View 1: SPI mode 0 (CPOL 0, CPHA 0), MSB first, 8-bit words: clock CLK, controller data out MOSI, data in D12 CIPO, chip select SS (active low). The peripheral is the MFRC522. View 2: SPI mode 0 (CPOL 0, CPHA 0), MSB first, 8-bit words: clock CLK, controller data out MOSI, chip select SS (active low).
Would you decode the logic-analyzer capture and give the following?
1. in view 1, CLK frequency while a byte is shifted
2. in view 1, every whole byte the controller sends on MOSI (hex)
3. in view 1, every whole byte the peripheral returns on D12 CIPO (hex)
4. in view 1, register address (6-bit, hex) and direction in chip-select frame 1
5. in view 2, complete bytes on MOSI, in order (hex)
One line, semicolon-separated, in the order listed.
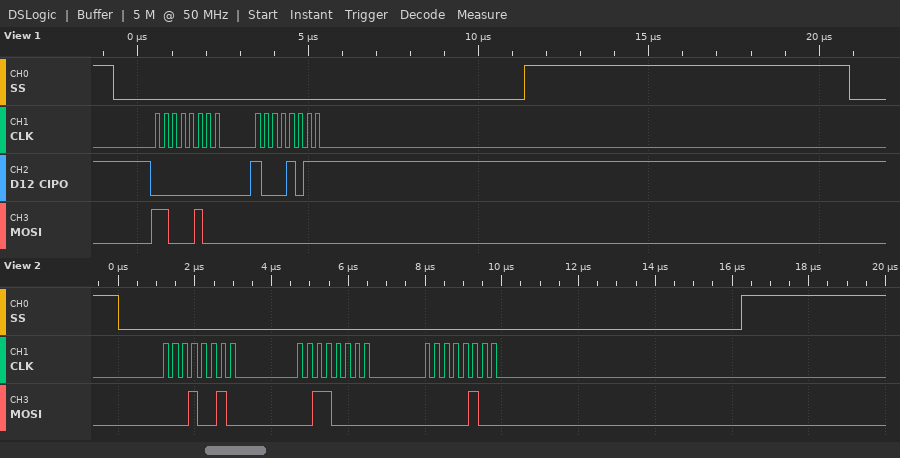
4 MHz; 0xC4 0x00; 0x00 0x8B; 0x22 read; 12 30 04
